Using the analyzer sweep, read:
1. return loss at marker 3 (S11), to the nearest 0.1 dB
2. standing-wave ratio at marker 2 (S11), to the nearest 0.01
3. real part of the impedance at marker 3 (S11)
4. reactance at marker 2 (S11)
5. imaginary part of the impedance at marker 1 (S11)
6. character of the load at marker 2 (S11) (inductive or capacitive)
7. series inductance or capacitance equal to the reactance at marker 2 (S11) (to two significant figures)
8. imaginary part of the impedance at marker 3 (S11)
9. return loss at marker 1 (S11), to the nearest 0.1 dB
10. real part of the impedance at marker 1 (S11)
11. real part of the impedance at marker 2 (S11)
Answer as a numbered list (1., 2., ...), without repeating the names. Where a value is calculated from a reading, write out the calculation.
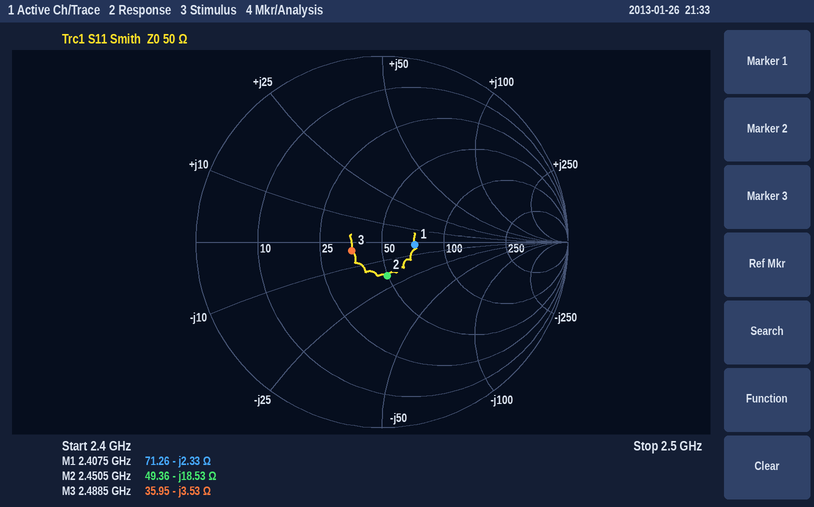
1. 15.5 dB
2. 1.45
3. 35.95 Ω
4. -18.53 Ω
5. -2.33 Ω
6. capacitive
7. C = 1/(2π × 2.4505 GHz × 18.53 Ω) ≈ 3.5 pF
8. -3.53 Ω
9. 15.1 dB
10. 71.26 Ω
11. 49.36 Ω
